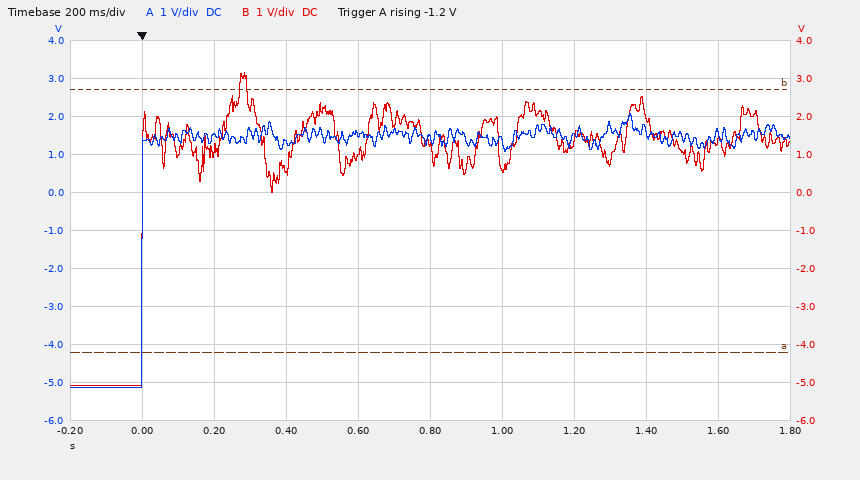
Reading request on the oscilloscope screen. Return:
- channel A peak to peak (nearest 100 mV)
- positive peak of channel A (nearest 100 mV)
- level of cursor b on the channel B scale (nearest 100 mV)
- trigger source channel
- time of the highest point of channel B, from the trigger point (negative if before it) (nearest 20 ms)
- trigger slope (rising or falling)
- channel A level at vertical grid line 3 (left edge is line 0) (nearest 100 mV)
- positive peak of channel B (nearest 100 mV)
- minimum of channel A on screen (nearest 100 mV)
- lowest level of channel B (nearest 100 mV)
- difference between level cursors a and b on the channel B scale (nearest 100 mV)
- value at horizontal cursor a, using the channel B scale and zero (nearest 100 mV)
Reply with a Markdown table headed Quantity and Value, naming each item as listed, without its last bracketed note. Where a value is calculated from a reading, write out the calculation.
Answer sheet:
| Quantity | Value |
|---|---|
| channel A peak to peak | 2.1 V − (-5.1 V) = 7.2 V |
| positive peak of channel A | 2.1 V |
| level of cursor b on the channel B scale | 2.7 V |
| trigger source channel | channel A |
| time of the highest point of channel B, from the trigger point (negative if before it) | +280 ms |
| trigger slope | rising |
| channel A level at vertical grid line 3 (left edge is line 0) | 1.3 V |
| positive peak of channel B | 3.2 V |
| minimum of channel A on screen | -5.1 V |
| lowest level of channel B | -5.1 V |
| difference between level cursors a and b on the channel B scale | 6.9 V |
| value at horizontal cursor a, using the channel B scale and zero | -4.2 V |
